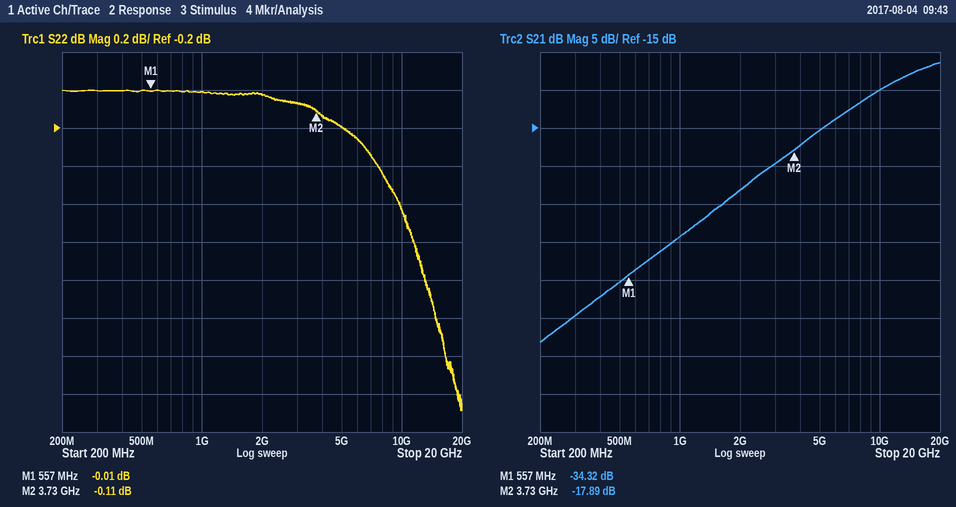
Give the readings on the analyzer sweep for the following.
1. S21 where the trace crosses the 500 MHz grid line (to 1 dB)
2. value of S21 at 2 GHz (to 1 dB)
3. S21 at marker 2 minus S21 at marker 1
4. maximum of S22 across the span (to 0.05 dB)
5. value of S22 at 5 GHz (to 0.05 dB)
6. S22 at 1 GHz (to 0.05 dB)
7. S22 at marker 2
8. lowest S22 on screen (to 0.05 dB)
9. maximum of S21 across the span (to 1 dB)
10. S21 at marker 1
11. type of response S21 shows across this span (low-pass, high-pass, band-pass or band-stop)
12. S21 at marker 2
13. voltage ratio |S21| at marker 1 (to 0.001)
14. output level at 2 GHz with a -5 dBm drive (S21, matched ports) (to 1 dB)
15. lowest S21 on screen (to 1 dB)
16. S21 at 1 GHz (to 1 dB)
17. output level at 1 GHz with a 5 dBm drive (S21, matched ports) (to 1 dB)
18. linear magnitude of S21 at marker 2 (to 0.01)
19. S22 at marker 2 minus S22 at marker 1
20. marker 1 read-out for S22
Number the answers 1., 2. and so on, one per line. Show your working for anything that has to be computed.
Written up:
1. -35 dB
2. -23 dB
3. -17.89 − (-34.32) = 16.43 dB
4. 0.00 dB
5. -0.20 dB
6. 0.00 dB
7. -0.11 dB
8. -1.70 dB
9. -6 dB
10. -34.32 dB
11. high-pass
12. -17.89 dB
13. 10^(-34.32/20) ≈ 0.019
14. -5 dBm + (-23 dB) = -28 dBm
15. -43 dB
16. -29 dB
17. 5 dBm + (-29 dB) = -24 dBm
18. 10^(-17.89/20) ≈ 0.13
19. -0.11 − (-0.01) = -0.10 dB
20. -0.01 dB
